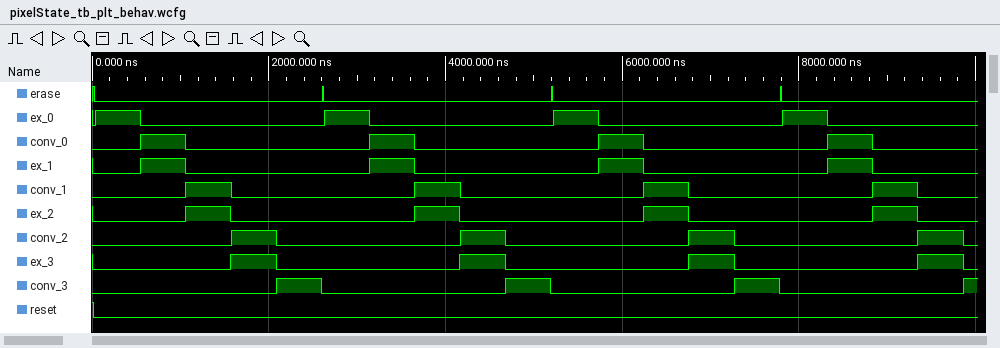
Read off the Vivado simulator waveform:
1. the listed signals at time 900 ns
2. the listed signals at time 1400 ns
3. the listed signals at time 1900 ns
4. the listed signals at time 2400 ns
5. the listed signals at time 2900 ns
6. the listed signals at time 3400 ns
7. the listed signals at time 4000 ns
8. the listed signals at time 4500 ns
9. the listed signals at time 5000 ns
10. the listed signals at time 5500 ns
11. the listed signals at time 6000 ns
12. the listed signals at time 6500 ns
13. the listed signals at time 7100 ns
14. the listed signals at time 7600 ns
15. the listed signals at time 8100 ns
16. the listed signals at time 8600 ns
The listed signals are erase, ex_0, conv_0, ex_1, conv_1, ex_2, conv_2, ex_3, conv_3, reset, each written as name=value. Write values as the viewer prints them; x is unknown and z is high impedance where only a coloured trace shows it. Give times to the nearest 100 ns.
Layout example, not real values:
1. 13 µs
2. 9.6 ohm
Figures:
1. erase=0, ex_0=0, conv_0=1, ex_1=1, conv_1=0, ex_2=0, conv_2=0, ex_3=0, conv_3=0, reset=0
2. erase=0, ex_0=0, conv_0=0, ex_1=0, conv_1=1, ex_2=1, conv_2=0, ex_3=0, conv_3=0, reset=0
3. erase=0, ex_0=0, conv_0=0, ex_1=0, conv_1=0, ex_2=0, conv_2=1, ex_3=1, conv_3=0, reset=0
4. erase=0, ex_0=0, conv_0=0, ex_1=0, conv_1=0, ex_2=0, conv_2=0, ex_3=0, conv_3=1, reset=0
5. erase=0, ex_0=1, conv_0=0, ex_1=0, conv_1=0, ex_2=0, conv_2=0, ex_3=0, conv_3=0, reset=0
6. erase=0, ex_0=0, conv_0=1, ex_1=1, conv_1=0, ex_2=0, conv_2=0, ex_3=0, conv_3=0, reset=0
7. erase=0, ex_0=0, conv_0=0, ex_1=0, conv_1=1, ex_2=1, conv_2=0, ex_3=0, conv_3=0, reset=0
8. erase=0, ex_0=0, conv_0=0, ex_1=0, conv_1=0, ex_2=0, conv_2=1, ex_3=1, conv_3=0, reset=0
9. erase=0, ex_0=0, conv_0=0, ex_1=0, conv_1=0, ex_2=0, conv_2=0, ex_3=0, conv_3=1, reset=0
10. erase=0, ex_0=1, conv_0=0, ex_1=0, conv_1=0, ex_2=0, conv_2=0, ex_3=0, conv_3=0, reset=0
11. erase=0, ex_0=0, conv_0=1, ex_1=1, conv_1=0, ex_2=0, conv_2=0, ex_3=0, conv_3=0, reset=0
12. erase=0, ex_0=0, conv_0=0, ex_1=0, conv_1=1, ex_2=1, conv_2=0, ex_3=0, conv_3=0, reset=0
13. erase=0, ex_0=0, conv_0=0, ex_1=0, conv_1=0, ex_2=0, conv_2=1, ex_3=1, conv_3=0, reset=0
14. erase=0, ex_0=0, conv_0=0, ex_1=0, conv_1=0, ex_2=0, conv_2=0, ex_3=0, conv_3=1, reset=0
15. erase=0, ex_0=1, conv_0=0, ex_1=0, conv_1=0, ex_2=0, conv_2=0, ex_3=0, conv_3=0, reset=0
16. erase=0, ex_0=0, conv_0=1, ex_1=1, conv_1=0, ex_2=0, conv_2=0, ex_3=0, conv_3=0, reset=0
